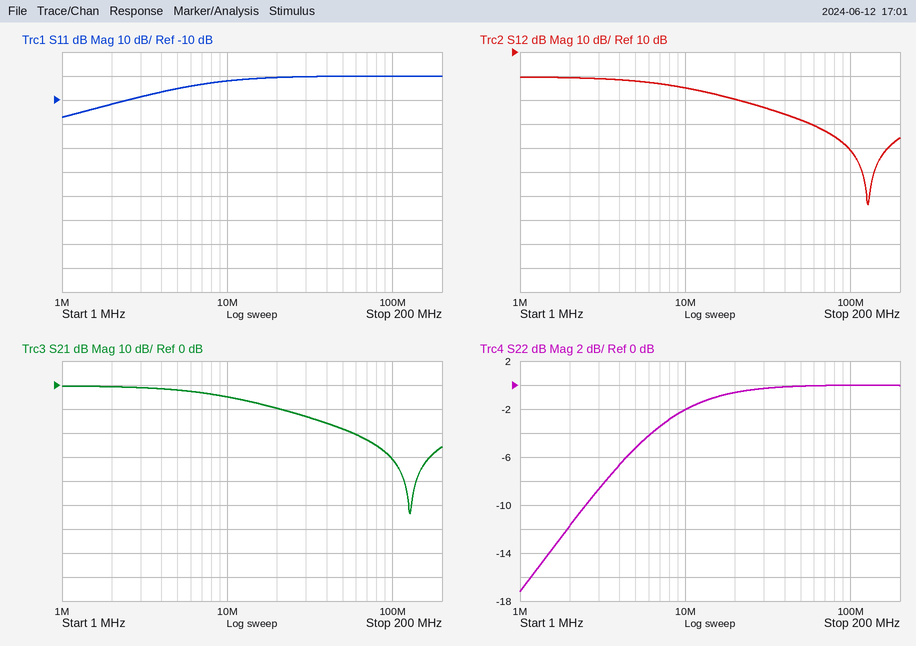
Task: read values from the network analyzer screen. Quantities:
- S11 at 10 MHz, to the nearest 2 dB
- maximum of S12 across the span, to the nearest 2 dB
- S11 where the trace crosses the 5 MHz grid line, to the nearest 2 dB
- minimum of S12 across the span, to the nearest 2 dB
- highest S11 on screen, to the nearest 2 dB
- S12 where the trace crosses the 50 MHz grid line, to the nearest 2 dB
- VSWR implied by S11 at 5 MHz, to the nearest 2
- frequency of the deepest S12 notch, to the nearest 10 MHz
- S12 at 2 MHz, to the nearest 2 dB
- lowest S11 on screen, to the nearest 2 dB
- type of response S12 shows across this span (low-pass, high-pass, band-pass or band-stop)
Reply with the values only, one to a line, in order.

-2 dB
0 dB
-6 dB
-54 dB
0 dB
-18 dB
4
130 MHz
0 dB
-18 dB
low-pass
